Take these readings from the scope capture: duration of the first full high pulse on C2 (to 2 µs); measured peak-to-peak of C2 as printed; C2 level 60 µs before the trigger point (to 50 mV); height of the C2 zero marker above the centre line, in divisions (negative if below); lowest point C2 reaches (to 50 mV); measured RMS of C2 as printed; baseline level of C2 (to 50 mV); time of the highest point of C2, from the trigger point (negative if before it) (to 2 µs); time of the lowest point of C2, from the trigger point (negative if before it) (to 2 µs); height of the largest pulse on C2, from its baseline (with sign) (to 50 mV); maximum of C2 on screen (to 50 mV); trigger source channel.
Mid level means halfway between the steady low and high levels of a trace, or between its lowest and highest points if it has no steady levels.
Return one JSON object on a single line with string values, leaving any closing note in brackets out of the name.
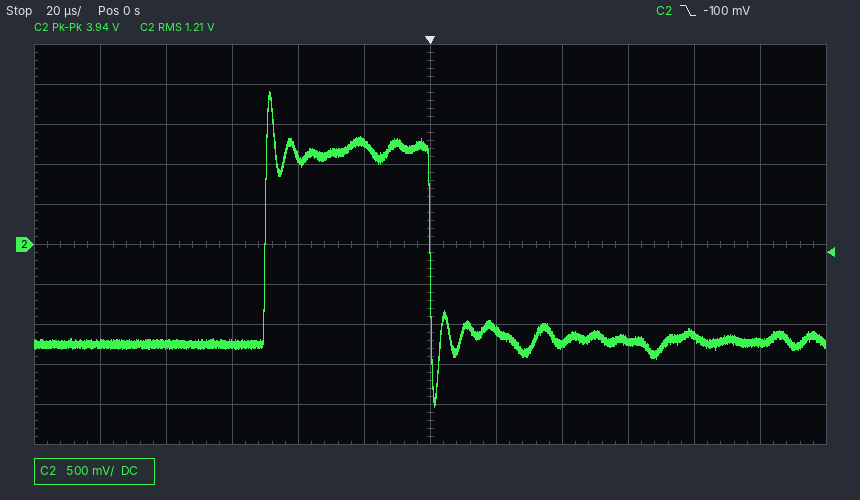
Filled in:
{"duration of the first full high pulse on C2": "50 µs", "measured peak-to-peak of C2 as printed": "3.94 V", "C2 level 60 µs before the trigger point": "-1.25 V", "height of the C2 zero marker above the centre line, in divisions": "0.0 div", "lowest point C2 reaches": "-2.00 V", "measured RMS of C2 as printed": "1.21 V", "baseline level of C2": "-1.25 V", "time of the highest point of C2, from the trigger point (negative if before it)": "-48 µs", "time of the lowest point of C2, from the trigger point (negative if before it)": "+2 µs", "height of the largest pulse on C2, from its baseline (with sign)": "+3.15 V", "maximum of C2 on screen": "1.90 V", "trigger source channel": "C2"}
